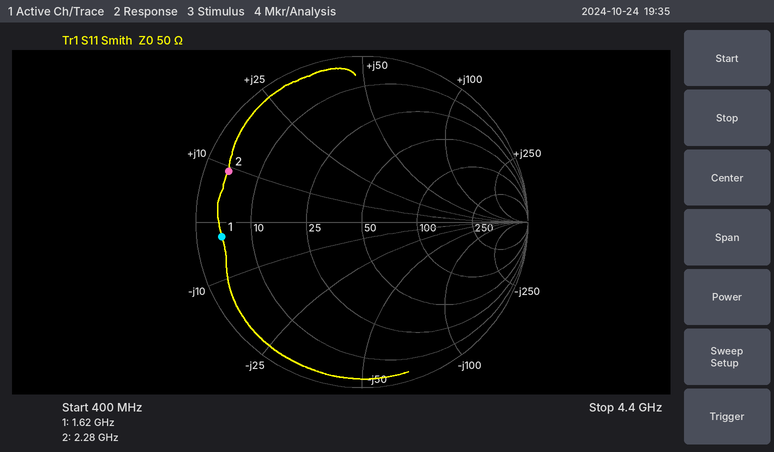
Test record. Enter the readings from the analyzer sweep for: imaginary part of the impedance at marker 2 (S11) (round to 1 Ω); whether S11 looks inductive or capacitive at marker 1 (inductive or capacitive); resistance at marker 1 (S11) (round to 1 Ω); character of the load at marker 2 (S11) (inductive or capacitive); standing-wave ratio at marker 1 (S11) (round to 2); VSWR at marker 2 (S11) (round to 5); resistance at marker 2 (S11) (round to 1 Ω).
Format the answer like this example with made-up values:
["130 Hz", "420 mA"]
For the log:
["+9 Ω", "capacitive", "4 Ω", "inductive", "12", "15", "4 Ω"]
